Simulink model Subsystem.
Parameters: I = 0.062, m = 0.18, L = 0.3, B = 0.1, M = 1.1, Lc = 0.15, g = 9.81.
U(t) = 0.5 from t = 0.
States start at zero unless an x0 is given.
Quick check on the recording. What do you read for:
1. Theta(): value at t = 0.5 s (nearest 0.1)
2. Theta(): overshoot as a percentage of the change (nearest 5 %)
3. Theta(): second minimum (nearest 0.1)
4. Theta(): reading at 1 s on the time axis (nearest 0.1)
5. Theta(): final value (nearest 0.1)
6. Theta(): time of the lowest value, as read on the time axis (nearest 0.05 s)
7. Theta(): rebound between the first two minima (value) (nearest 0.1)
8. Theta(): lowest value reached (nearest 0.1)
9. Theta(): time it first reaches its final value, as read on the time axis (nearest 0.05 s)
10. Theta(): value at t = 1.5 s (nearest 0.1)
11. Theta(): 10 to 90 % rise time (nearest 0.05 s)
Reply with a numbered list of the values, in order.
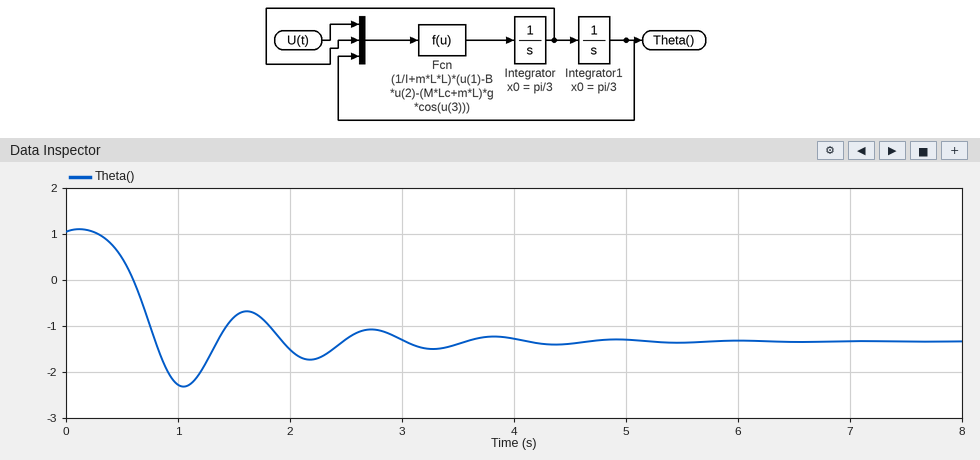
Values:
1. 0.5
2. 40 %
3. -1.7
4. -2.3
5. -1.3
6. 1.05 s
7. -0.7
8. -2.3
9. 0.80 s
10. -0.8
11. 0.35 s
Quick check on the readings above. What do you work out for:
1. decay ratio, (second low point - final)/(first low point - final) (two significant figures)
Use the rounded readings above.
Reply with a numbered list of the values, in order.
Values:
1. 0.40
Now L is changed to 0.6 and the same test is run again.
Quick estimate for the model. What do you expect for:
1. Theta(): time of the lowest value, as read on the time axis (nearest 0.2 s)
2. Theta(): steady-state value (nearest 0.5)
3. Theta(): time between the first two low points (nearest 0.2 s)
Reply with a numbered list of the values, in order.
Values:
1. 0.8 s
2. -1.5
3. 1.0 s
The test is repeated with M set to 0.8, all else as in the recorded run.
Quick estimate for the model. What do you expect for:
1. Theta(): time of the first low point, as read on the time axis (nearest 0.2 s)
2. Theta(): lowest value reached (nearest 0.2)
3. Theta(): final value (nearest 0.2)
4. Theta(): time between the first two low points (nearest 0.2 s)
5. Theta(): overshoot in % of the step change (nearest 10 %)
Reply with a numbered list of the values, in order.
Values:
1. 1.4 s
2. -2.2
3. -1.2
4. 1.2 s
5. 40 %
